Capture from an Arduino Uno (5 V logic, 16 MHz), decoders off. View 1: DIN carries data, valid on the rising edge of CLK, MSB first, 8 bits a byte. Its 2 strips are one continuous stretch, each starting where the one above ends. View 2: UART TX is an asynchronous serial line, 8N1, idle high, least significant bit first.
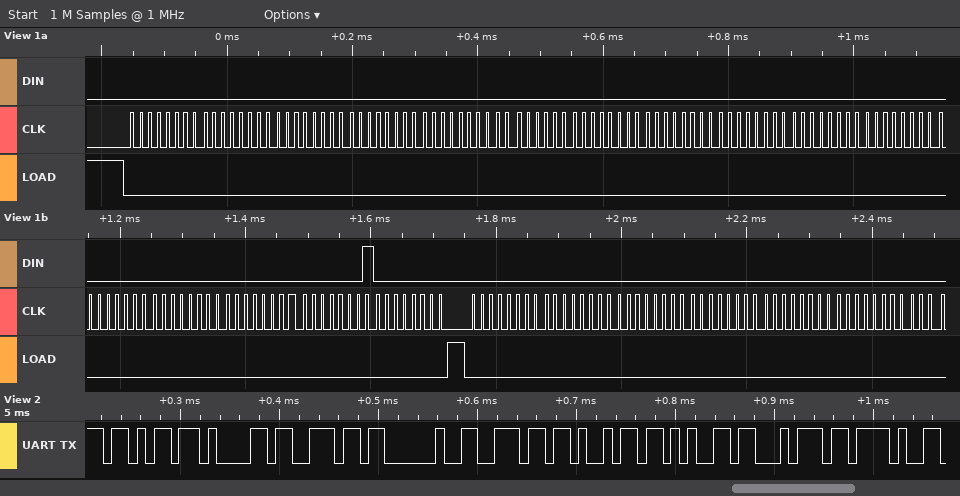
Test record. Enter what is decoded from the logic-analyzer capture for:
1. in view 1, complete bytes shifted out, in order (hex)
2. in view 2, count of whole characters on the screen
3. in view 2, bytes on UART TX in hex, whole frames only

00 00 00 00 00 00 00 00 00 00 00 00 00 00 01 00 00 00 00 00 00 00
9
0x6B 0x61 0x6E 0x20 0x6E 0x69 0x65 0x74 0x2F
